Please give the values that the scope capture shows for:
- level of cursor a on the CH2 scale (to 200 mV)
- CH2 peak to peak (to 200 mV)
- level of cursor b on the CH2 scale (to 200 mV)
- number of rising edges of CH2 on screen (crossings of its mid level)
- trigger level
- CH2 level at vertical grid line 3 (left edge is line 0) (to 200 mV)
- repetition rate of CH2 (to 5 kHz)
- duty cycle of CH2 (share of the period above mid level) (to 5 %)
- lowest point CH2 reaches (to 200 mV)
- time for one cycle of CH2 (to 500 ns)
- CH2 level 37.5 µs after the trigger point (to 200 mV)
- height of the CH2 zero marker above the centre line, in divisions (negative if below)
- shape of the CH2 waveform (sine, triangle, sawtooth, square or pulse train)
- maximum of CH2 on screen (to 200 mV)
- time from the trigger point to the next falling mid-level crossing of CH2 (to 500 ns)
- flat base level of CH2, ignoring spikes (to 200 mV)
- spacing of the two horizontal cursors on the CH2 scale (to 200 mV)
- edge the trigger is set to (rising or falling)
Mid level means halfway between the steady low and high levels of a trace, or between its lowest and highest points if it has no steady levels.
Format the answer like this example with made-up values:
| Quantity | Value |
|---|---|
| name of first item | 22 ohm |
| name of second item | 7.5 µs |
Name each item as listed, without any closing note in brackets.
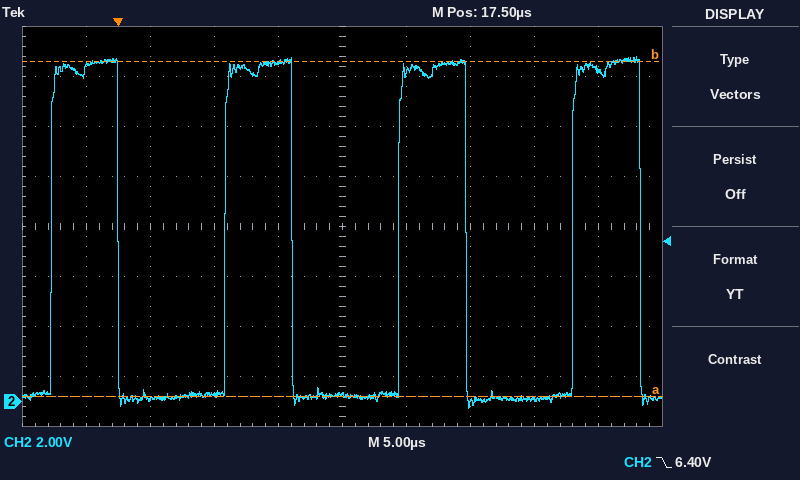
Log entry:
| Quantity | Value |
|---|---|
| level of cursor a on the CH2 scale | 200 mV |
| CH2 peak to peak | 14.0 V |
| level of cursor b on the CH2 scale | 13.6 V |
| number of rising edges of CH2 on screen | 4 |
| trigger level | 6.40 V |
| CH2 level at vertical grid line 3 (left edge is line 0) | 200 mV |
| repetition rate of CH2 | 75 kHz |
| duty cycle of CH2 (share of the period above mid level) | 40 % |
| lowest point CH2 reaches | -200 mV |
| time for one cycle of CH2 | 13.5 µs |
| CH2 level 37.5 µs after the trigger point | 13.2 V |
| height of the CH2 zero marker above the centre line, in divisions | -3.5 div |
| shape of the CH2 waveform | pulse train |
| maximum of CH2 on screen | 13.8 V |
| time from the trigger point to the next falling mid-level crossing of CH2 | 13.5 µs |
| flat base level of CH2, ignoring spikes | 200 mV |
| spacing of the two horizontal cursors on the CH2 scale | 13.4 V |
| edge the trigger is set to | falling |
